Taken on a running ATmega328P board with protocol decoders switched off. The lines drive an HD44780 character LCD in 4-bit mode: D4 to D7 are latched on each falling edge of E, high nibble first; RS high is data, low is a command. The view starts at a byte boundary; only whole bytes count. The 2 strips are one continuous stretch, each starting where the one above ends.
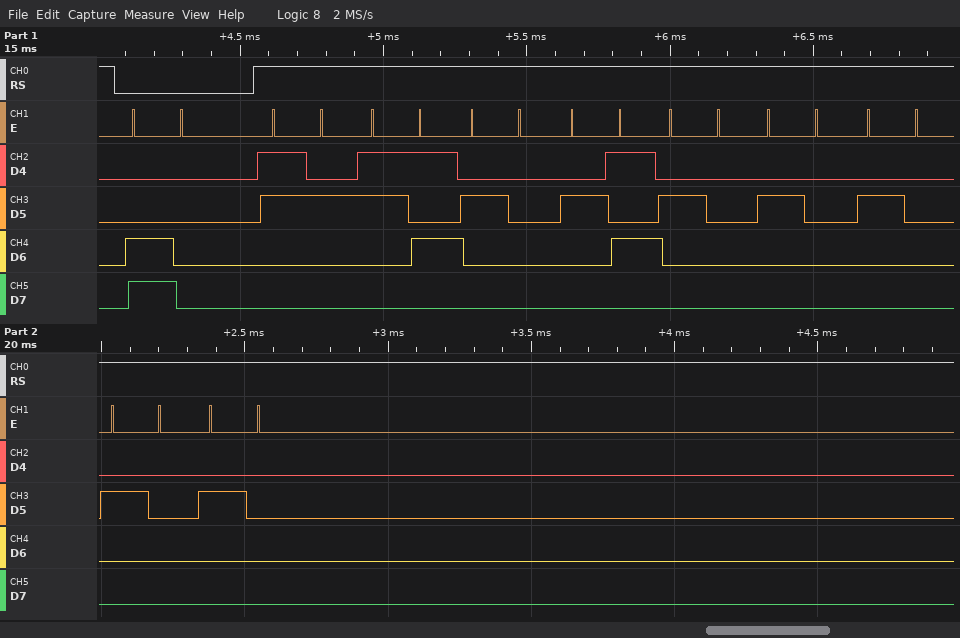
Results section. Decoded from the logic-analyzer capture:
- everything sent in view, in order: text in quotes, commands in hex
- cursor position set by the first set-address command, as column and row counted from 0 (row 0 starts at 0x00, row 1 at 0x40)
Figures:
0xC0 "25 %     "
column 0, row 1
